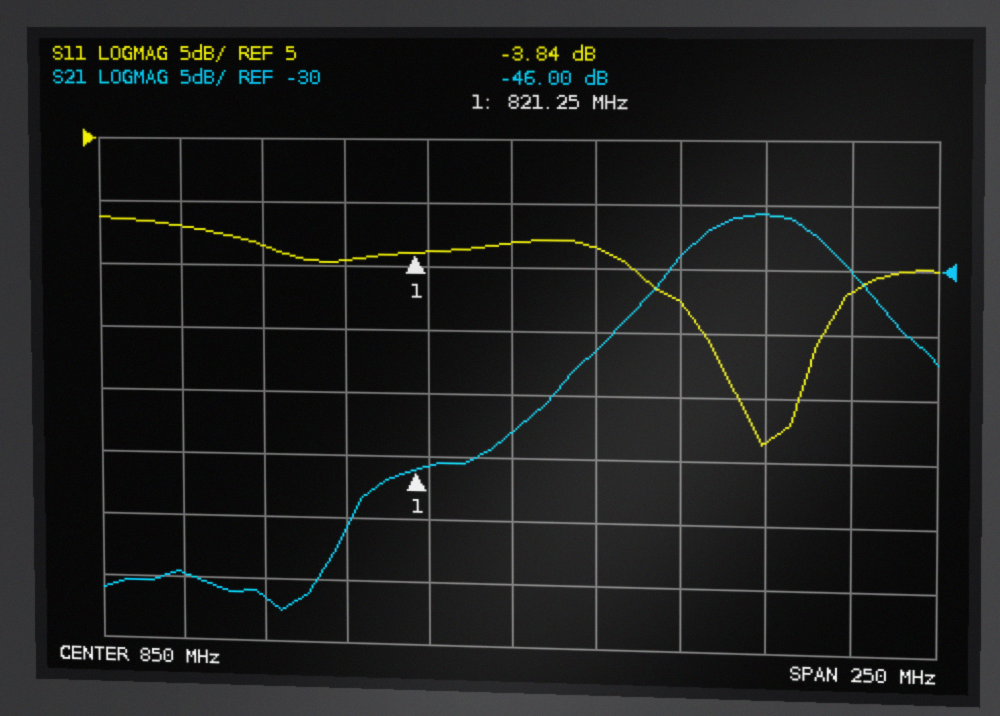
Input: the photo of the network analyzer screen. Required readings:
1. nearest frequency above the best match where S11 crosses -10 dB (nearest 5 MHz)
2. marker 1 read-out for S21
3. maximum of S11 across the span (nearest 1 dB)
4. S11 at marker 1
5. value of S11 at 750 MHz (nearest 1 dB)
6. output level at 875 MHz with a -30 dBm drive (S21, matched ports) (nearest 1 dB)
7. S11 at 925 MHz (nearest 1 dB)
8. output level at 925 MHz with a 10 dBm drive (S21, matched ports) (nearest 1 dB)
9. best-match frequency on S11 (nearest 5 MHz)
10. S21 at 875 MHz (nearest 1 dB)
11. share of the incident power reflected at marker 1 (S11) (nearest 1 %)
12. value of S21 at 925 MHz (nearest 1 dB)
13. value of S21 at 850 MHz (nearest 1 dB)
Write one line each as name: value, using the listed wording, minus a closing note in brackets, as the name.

nearest frequency above the best match where S11 crosses -10 dB: 940 MHz
marker 1 read-out for S21: -46.00 dB
maximum of S11 across the span: -1 dB
S11 at marker 1: -3.84 dB
value of S11 at 750 MHz: -2 dB
output level at 875 MHz with a -30 dBm drive (S21, matched ports): -66 dBm
S11 at 925 MHz: -18 dB
output level at 925 MHz with a 10 dBm drive (S21, matched ports): -16 dBm
best-match frequency on S11: 925 MHz
S21 at 875 MHz: -36 dB
share of the incident power reflected at marker 1 (S11): 41 %
value of S21 at 925 MHz: -26 dB
value of S21 at 850 MHz: -43 dB
